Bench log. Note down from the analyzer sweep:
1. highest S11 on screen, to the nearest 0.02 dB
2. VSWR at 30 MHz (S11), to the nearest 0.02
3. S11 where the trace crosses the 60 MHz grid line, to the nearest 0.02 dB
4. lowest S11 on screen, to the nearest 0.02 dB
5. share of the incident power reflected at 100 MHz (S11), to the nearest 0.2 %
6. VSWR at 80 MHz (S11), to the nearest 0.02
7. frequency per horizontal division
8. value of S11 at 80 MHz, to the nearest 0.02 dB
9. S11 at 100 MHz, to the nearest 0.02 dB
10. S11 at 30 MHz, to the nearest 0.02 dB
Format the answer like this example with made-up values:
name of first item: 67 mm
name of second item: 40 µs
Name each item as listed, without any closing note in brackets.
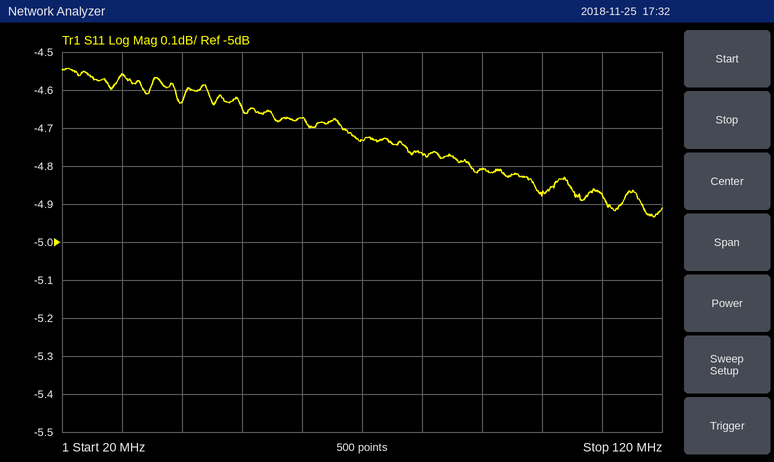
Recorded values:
highest S11 on screen, to the nearest 0.02 dB: -4.54 dB
VSWR at 30 MHz (S11), to the nearest 0.02: 3.90
S11 where the trace crosses the 60 MHz grid line, to the nearest 0.02 dB: -4.68 dB
lowest S11 on screen, to the nearest 0.02 dB: -4.94 dB
share of the incident power reflected at 100 MHz (S11), to the nearest 0.2 %: 32.6 %
VSWR at 80 MHz (S11), to the nearest 0.02: 3.74
frequency per horizontal division: 10 MHz
value of S11 at 80 MHz, to the nearest 0.02 dB: -4.76 dB
S11 at 100 MHz, to the nearest 0.02 dB: -4.88 dB
S11 at 30 MHz, to the nearest 0.02 dB: -4.56 dB
